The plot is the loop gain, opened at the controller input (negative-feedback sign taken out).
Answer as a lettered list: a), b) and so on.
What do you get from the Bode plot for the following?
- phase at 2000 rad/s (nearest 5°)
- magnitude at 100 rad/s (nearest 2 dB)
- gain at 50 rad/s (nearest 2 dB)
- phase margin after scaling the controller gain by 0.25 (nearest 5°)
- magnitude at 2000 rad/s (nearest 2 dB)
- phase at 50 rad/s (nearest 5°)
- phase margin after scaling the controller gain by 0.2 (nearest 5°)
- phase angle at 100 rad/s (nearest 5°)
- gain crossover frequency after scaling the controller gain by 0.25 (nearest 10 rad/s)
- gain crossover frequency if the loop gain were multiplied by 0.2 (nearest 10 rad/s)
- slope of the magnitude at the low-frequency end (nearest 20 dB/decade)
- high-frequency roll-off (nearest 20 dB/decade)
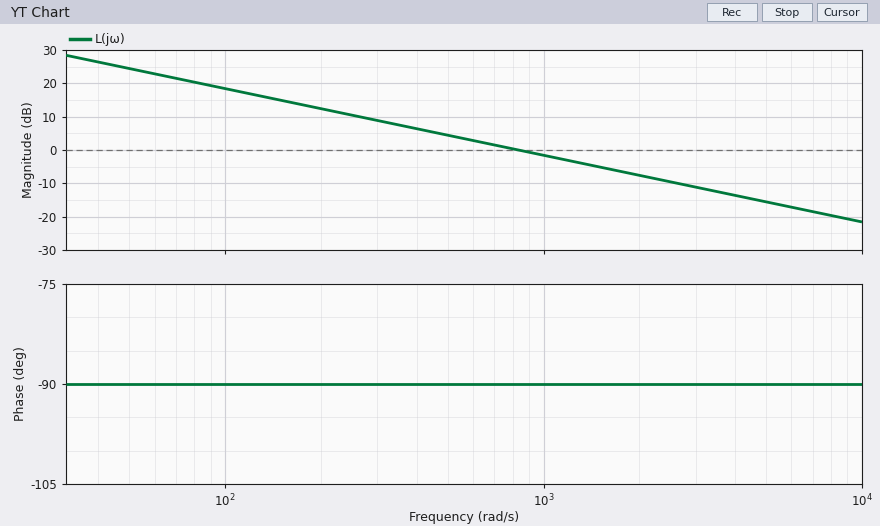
a) -90°
b) 18 dB
c) 24 dB
d) 90°
e) -8 dB
f) -90°
g) 90°
h) -90°
i) 210 rad/s
j) 170 rad/s
k) -20 dB/decade
l) -20 dB/decade
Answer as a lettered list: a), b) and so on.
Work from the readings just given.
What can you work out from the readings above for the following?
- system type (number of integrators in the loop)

a) 1
